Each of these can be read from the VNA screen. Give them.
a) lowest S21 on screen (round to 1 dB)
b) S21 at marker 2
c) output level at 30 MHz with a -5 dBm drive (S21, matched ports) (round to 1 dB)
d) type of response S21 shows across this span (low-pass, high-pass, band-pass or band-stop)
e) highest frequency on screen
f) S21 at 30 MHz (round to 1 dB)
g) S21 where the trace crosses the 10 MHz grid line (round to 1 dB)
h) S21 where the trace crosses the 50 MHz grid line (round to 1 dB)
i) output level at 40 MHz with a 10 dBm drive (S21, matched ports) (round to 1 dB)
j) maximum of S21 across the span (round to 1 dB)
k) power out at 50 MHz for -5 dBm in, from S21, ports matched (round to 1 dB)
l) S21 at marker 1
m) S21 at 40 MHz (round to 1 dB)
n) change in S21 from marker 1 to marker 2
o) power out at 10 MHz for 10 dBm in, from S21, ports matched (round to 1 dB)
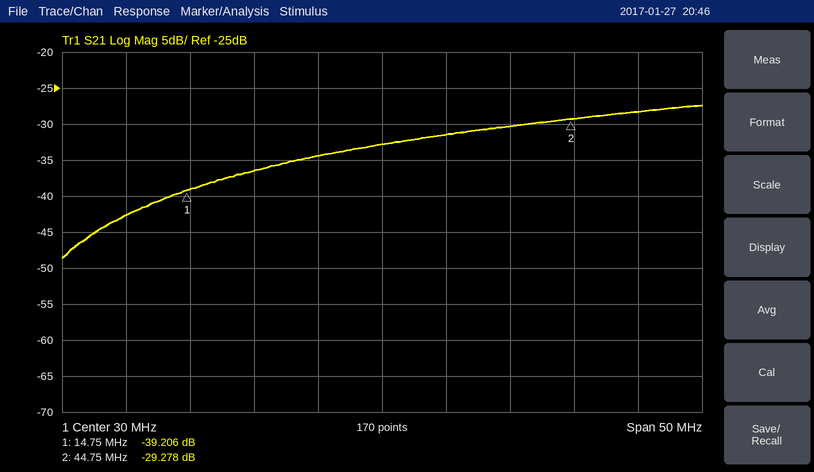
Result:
-49 dB
-29.278 dB
-38 dBm
high-pass
55 MHz
-33 dB
-43 dB
-28 dB
-20 dBm
-27 dB
-33 dBm
-39.206 dB
-30 dB
9.928 dB
-33 dBm
